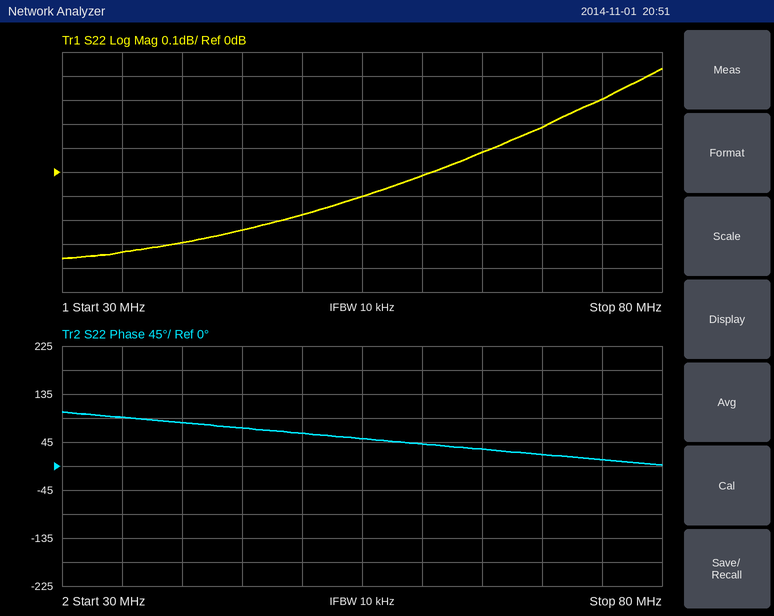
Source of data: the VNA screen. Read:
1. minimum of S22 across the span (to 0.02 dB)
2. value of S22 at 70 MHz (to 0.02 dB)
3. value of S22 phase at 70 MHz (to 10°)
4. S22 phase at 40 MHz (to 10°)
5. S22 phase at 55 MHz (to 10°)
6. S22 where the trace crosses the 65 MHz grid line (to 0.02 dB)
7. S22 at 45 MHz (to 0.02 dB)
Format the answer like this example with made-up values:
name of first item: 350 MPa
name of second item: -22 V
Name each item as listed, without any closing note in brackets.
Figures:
minimum of S22 across the span: -0.36 dB
value of S22 at 70 MHz: 0.18 dB
value of S22 phase at 70 MHz: 20°
S22 phase at 40 MHz: 80°
S22 phase at 55 MHz: 50°
S22 where the trace crosses the 65 MHz grid line: 0.08 dB
S22 at 45 MHz: -0.24 dB
